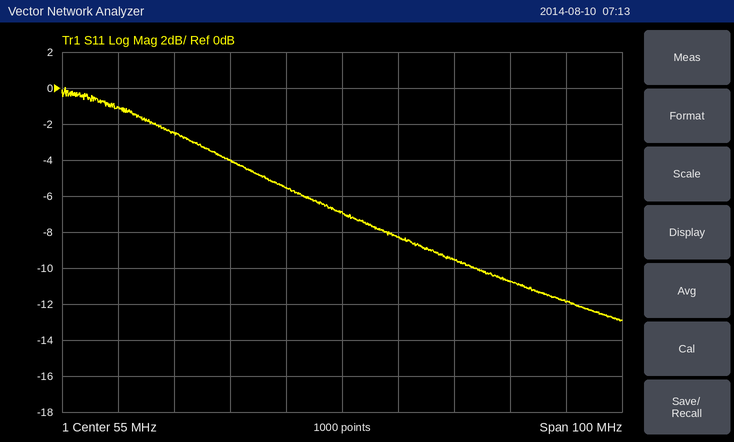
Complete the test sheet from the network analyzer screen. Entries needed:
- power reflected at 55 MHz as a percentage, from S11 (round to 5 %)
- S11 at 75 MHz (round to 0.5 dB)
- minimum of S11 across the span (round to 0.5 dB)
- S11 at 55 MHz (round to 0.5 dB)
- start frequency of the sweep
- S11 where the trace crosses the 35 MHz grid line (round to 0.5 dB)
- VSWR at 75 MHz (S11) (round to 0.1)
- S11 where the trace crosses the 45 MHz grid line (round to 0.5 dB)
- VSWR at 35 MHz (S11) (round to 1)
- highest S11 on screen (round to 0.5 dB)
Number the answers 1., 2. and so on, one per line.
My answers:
1. 20 %
2. -9.5 dB
3. -13.0 dB
4. -7.0 dB
5. 5 MHz
6. -4.0 dB
7. 2.0
8. -5.5 dB
9. 4
10. 0.0 dB
